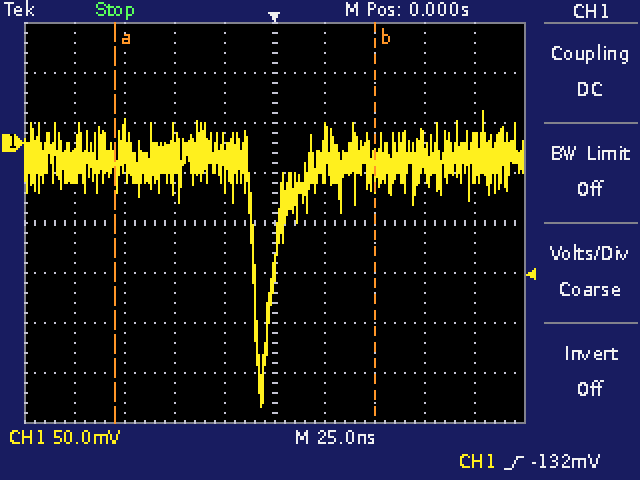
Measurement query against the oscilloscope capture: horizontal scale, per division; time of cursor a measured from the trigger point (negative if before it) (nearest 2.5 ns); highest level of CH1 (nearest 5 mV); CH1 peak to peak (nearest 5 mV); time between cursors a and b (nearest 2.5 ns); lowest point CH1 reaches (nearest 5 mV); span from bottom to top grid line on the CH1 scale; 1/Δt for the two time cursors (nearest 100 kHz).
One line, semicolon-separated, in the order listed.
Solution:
25 ns; -80.0 ns; 30 mV; 295 mV; 130.0 ns; -265 mV; 400 mV; 7.7 MHz
